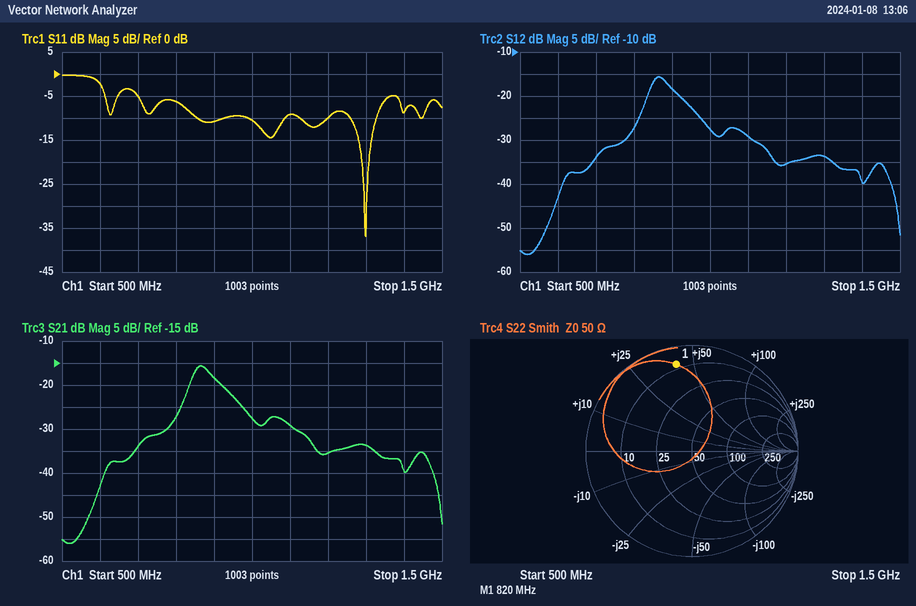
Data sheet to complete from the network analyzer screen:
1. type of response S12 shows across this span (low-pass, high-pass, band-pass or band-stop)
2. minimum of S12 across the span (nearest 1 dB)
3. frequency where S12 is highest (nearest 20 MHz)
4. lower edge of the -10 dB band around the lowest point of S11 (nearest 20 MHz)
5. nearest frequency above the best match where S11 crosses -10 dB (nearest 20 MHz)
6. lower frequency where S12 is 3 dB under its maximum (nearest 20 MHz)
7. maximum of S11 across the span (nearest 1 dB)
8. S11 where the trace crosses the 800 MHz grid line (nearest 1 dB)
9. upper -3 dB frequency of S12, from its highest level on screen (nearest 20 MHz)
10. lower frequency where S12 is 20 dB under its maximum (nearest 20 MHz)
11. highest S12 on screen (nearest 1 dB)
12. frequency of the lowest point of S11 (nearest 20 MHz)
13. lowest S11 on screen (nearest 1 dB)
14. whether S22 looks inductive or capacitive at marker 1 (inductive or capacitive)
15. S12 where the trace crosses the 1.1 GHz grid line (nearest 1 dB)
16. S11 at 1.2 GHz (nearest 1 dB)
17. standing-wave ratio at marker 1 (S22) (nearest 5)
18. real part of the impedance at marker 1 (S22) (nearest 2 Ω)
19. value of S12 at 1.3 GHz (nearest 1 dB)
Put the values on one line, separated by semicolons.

band-pass; -56 dB; 860 MHz; 1.26 GHz; 1.32 GHz; 840 MHz; 0 dB; -6 dB; 900 MHz; 680 MHz; -16 dB; 1.30 GHz; -37 dB; inductive; -29 dB; -10 dB; 10; 8 Ω; -34 dB
